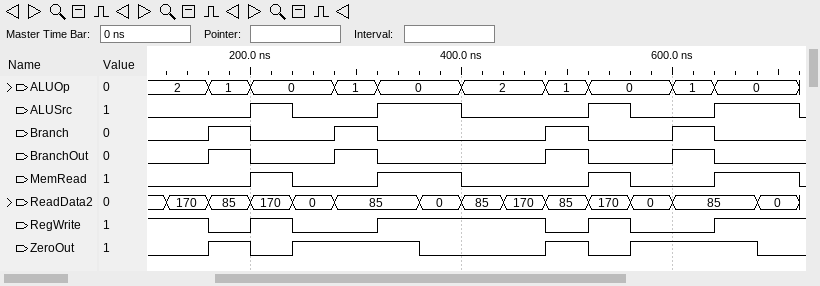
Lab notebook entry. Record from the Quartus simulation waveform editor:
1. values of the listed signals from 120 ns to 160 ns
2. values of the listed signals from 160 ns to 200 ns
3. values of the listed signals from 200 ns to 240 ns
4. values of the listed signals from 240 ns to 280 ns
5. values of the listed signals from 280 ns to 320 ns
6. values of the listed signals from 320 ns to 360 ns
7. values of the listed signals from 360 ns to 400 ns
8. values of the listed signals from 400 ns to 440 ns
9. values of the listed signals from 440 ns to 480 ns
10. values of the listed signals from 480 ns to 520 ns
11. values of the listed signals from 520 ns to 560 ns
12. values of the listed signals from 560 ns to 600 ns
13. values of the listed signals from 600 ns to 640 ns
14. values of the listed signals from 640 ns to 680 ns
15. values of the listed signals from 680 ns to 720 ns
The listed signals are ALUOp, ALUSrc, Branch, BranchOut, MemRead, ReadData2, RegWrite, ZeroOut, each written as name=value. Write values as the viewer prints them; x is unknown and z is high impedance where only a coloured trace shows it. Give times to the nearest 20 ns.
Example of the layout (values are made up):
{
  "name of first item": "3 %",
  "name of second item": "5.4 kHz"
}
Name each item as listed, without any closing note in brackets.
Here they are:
{
  "values of the listed signals from 120 ns to 160 ns": "ALUOp=2, ALUSrc=0, Branch=0, BranchOut=0, MemRead=0, ReadData2=170, RegWrite=1, ZeroOut=0",
  "values of the listed signals from 160 ns to 200 ns": "ALUOp=1, ALUSrc=0, Branch=1, BranchOut=1, MemRead=0, ReadData2=85, RegWrite=0, ZeroOut=1",
  "values of the listed signals from 200 ns to 240 ns": "ALUOp=0, ALUSrc=1, Branch=0, BranchOut=0, MemRead=1, ReadData2=170, RegWrite=1, ZeroOut=0",
  "values of the listed signals from 240 ns to 280 ns": "ALUOp=0, ALUSrc=0, Branch=0, BranchOut=0, MemRead=0, ReadData2=0, RegWrite=0, ZeroOut=1",
  "values of the listed signals from 280 ns to 320 ns": "ALUOp=1, ALUSrc=0, Branch=1, BranchOut=1, MemRead=0, ReadData2=85, RegWrite=0, ZeroOut=1",
  "values of the listed signals from 320 ns to 360 ns": "ALUOp=0, ALUSrc=1, Branch=0, BranchOut=0, MemRead=1, ReadData2=85, RegWrite=1, ZeroOut=1",
  "values of the listed signals from 360 ns to 400 ns": "ALUOp=0, ALUSrc=1, Branch=0, BranchOut=0, MemRead=1, ReadData2=0, RegWrite=1, ZeroOut=0",
  "values of the listed signals from 400 ns to 440 ns": "ALUOp=2, ALUSrc=0, Branch=0, BranchOut=0, MemRead=0, ReadData2=85, RegWrite=1, ZeroOut=0",
  "values of the listed signals from 440 ns to 480 ns": "ALUOp=2, ALUSrc=0, Branch=0, BranchOut=0, MemRead=0, ReadData2=170, RegWrite=1, ZeroOut=0",
  "values of the listed signals from 480 ns to 520 ns": "ALUOp=1, ALUSrc=0, Branch=1, BranchOut=1, MemRead=0, ReadData2=85, RegWrite=0, ZeroOut=1",
  "values of the listed signals from 520 ns to 560 ns": "ALUOp=0, ALUSrc=1, Branch=0, BranchOut=0, MemRead=1, ReadData2=170, RegWrite=1, ZeroOut=0",
  "values of the listed signals from 560 ns to 600 ns": "ALUOp=0, ALUSrc=0, Branch=0, BranchOut=0, MemRead=0, ReadData2=0, RegWrite=0, ZeroOut=1",
  "values of the listed signals from 600 ns to 640 ns": "ALUOp=1, ALUSrc=0, Branch=1, BranchOut=1, MemRead=0, ReadData2=85, RegWrite=0, ZeroOut=1",
  "values of the listed signals from 640 ns to 680 ns": "ALUOp=0, ALUSrc=1, Branch=0, BranchOut=0, MemRead=1, ReadData2=85, RegWrite=1, ZeroOut=1",
  "values of the listed signals from 680 ns to 720 ns": "ALUOp=0, ALUSrc=1, Branch=0, BranchOut=0, MemRead=1, ReadData2=0, RegWrite=1, ZeroOut=0"
}
